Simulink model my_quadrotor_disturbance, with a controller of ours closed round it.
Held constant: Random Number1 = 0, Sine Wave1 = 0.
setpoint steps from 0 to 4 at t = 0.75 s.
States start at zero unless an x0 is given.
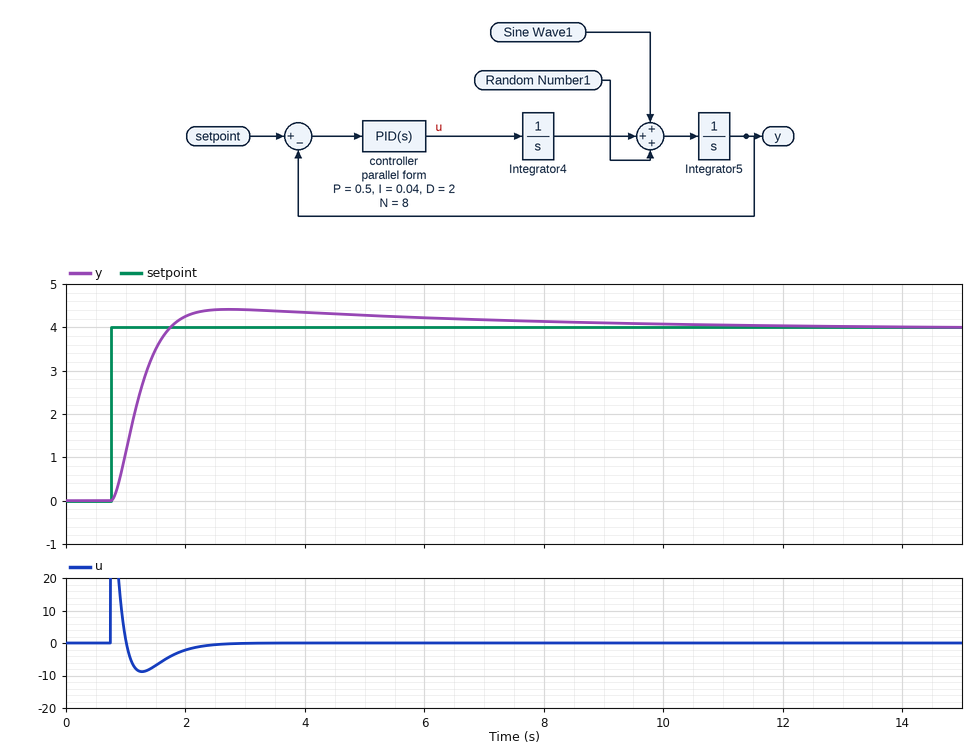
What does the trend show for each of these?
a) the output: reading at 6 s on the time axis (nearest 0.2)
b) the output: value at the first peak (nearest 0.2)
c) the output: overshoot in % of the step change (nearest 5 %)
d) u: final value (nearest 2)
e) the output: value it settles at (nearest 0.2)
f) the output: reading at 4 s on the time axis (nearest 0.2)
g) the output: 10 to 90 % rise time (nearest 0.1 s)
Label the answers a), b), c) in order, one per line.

a) 4.2
b) 4.4
c) 10 %
d) 0
e) 4.0
f) 4.4
g) 0.7 s
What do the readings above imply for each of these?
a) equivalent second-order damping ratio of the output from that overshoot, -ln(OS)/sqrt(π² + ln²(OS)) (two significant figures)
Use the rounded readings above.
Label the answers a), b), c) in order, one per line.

a) 0.59
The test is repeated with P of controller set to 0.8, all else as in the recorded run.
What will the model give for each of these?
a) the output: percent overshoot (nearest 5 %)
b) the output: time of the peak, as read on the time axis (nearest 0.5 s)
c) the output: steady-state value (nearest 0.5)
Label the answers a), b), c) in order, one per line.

a) 15 %
b) 2.5 s
c) 4.0
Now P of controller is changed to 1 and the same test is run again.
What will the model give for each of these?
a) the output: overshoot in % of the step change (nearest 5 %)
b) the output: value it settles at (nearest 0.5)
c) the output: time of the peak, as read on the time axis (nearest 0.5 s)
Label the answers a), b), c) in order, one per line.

a) 15 %
b) 4.0
c) 2.5 s
